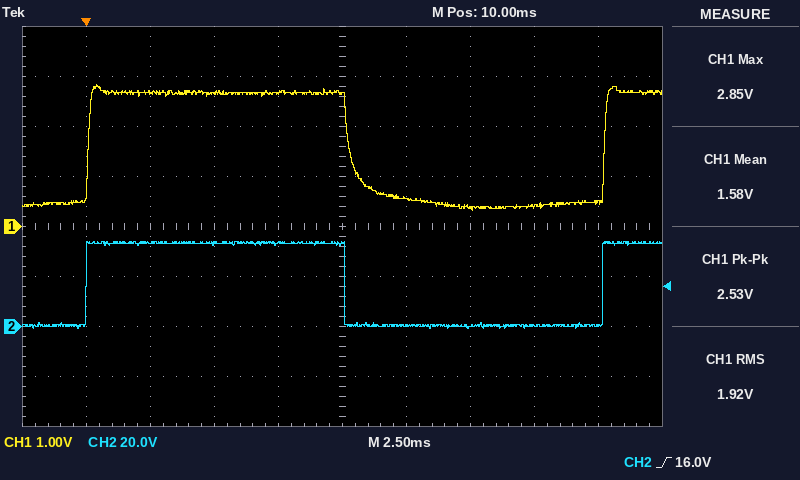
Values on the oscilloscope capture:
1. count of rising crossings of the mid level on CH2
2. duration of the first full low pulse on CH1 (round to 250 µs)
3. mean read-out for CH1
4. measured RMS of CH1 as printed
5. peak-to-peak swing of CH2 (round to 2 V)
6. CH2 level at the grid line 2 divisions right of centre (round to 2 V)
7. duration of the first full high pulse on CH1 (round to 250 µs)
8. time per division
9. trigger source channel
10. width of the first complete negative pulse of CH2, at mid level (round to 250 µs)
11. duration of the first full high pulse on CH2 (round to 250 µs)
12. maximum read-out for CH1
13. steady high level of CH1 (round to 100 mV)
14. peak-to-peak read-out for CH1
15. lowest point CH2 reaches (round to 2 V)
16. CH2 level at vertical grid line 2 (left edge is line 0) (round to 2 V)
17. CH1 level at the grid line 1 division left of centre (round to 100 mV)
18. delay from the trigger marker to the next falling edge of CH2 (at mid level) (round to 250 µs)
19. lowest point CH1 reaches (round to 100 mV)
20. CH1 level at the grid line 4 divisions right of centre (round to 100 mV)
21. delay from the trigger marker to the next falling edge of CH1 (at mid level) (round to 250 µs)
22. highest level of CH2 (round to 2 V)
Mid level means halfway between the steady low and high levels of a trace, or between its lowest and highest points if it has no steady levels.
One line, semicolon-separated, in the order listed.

2; 10.00 ms; 1.58 V; 1.92 V; 34 V; 0 V; 10.25 ms; 2.5 ms; CH2; 10.00 ms; 10.00 ms; 2.85 V; 2.7 V; 2.53 V; 0 V; 34 V; 2.7 V; 10.00 ms; 300 mV; 500 mV; 10.25 ms; 34 V
